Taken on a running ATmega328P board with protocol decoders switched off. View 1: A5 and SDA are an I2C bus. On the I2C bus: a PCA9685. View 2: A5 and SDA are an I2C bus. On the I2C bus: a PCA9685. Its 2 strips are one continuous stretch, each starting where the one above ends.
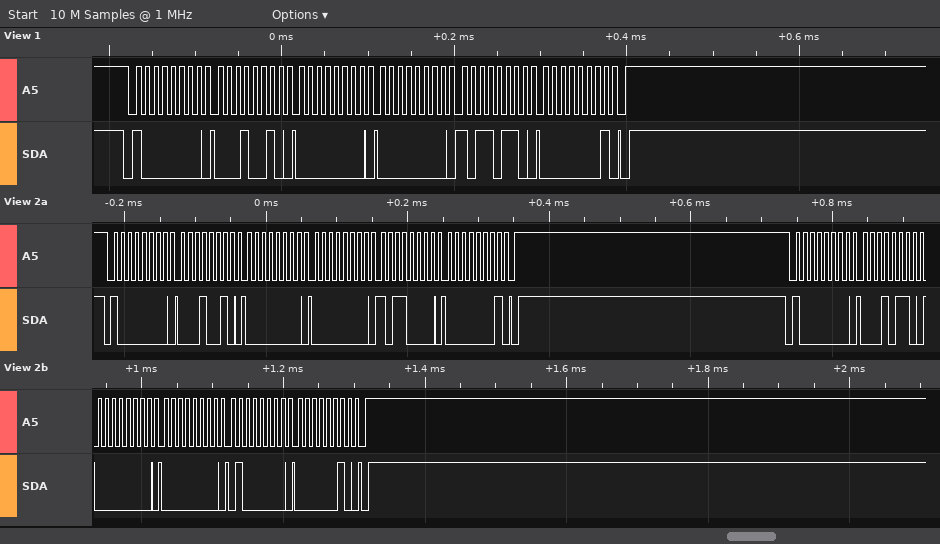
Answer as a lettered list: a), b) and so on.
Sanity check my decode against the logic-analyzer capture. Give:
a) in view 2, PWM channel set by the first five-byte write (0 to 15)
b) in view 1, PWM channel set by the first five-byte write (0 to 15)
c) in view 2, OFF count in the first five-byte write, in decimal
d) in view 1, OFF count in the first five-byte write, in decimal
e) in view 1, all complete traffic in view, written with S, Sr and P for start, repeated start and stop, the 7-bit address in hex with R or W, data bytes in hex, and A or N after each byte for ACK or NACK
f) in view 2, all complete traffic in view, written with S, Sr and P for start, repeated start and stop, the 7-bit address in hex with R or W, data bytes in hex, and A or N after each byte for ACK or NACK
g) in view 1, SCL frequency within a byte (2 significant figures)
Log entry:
a) 3
b) 3
c) 432
d) 438
e) S 40W A 12 A 00 A 00 A B6 A 01 A P
f) S 40W A 12 A 00 A 00 A B0 A 01 A P S 40W A 16 A 00 A 00 A 40 A 02 A P
g) 100 kHz
